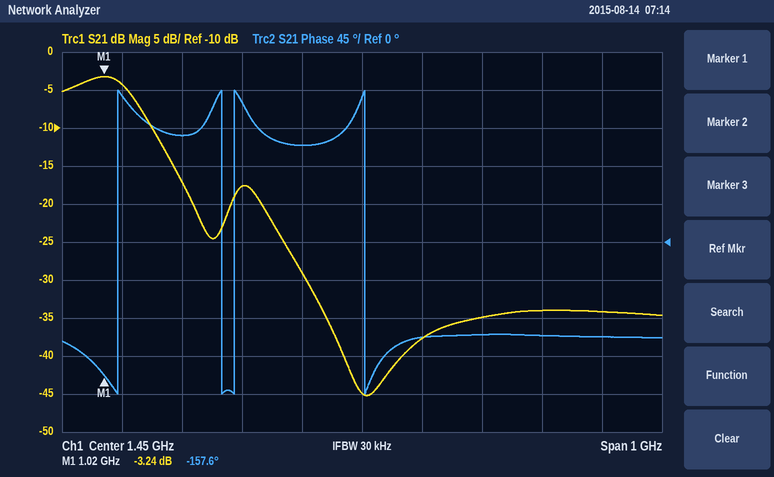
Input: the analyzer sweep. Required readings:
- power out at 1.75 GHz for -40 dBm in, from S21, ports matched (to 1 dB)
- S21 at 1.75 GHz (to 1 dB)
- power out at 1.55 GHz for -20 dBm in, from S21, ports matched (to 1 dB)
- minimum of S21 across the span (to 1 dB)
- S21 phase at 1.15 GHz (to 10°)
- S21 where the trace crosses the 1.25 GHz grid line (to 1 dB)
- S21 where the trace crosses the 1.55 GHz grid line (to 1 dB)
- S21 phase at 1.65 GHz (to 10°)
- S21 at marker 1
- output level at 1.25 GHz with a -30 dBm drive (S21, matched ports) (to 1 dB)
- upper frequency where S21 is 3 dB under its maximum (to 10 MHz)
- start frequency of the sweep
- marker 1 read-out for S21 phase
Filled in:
-74 dBm
-34 dB
-58 dBm
-45 dB
130°
-18 dB
-38 dB
-110°
-3.24 dB
-48 dBm
1.07 GHz
950 MHz
-157.6°
